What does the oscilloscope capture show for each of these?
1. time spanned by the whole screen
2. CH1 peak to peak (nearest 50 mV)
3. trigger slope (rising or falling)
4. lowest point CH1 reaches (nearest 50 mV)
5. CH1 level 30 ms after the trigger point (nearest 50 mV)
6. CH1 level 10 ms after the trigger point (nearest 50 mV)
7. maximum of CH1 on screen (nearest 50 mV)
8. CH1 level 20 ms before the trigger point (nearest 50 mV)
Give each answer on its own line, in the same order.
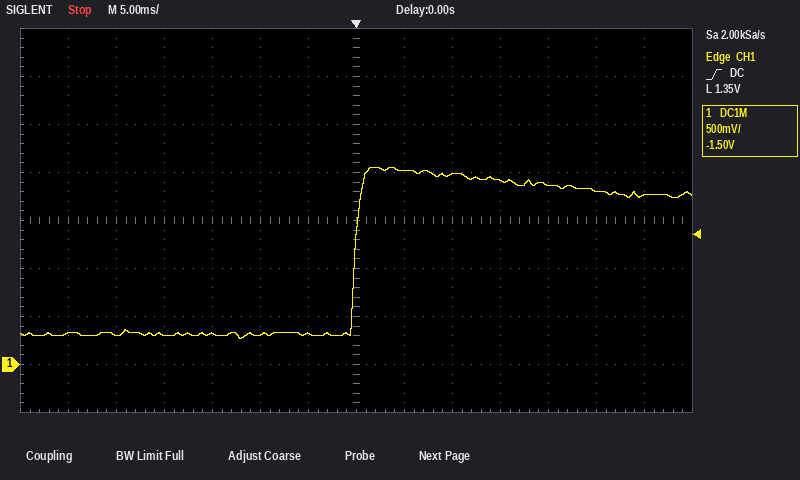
70 ms
1.80 V
rising
250 mV
1.75 V
2.00 V
2.05 V
300 mV
